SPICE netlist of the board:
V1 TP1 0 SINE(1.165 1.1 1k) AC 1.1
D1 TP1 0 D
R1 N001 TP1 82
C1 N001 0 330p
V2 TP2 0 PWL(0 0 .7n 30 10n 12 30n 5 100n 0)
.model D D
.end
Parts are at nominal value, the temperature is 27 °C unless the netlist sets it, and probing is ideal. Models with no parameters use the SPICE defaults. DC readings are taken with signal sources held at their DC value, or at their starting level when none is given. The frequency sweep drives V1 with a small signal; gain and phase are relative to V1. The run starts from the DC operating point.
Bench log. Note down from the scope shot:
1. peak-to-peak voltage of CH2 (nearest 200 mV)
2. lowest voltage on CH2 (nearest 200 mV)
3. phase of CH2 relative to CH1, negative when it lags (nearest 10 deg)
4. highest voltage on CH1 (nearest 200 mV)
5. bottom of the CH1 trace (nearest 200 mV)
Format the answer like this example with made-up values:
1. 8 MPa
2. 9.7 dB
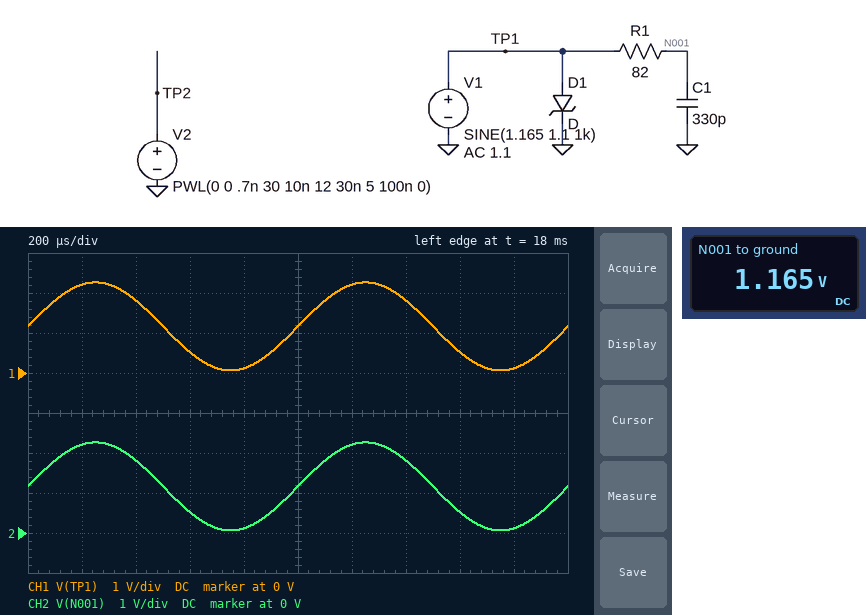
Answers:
1. 2.2 V
2. 0 V
3. 0 deg
4. 2.2 V
5. 0 V
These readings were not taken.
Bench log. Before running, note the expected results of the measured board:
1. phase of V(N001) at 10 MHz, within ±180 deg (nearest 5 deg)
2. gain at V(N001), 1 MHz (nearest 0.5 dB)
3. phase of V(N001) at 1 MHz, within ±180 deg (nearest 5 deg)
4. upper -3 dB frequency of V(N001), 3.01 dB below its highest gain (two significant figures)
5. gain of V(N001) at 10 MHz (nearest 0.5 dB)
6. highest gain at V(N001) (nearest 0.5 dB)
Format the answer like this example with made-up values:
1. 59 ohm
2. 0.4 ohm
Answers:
1. -60 deg
2. 0 dB
3. -10 deg
4. 5.9 MHz
5. -6.0 dB
6. 0 dB
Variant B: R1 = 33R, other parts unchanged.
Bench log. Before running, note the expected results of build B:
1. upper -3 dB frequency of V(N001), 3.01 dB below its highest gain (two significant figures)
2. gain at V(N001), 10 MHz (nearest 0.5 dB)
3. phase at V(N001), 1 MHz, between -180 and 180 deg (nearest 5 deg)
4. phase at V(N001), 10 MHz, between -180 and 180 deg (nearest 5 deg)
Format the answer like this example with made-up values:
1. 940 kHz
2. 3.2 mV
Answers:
1. 15 MHz
2. -1.5 dB
3. -5 deg
4. -35 deg
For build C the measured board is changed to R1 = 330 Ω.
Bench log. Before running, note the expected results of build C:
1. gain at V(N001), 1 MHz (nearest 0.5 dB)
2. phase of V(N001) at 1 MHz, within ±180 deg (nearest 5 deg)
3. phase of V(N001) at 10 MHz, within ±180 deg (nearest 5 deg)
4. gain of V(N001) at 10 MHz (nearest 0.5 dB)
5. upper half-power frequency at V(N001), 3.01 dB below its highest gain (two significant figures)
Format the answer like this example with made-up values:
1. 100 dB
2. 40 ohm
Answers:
1. -1.5 dB
2. -35 deg
3. -80 deg
4. -17.0 dB
5. 1.5 MHz
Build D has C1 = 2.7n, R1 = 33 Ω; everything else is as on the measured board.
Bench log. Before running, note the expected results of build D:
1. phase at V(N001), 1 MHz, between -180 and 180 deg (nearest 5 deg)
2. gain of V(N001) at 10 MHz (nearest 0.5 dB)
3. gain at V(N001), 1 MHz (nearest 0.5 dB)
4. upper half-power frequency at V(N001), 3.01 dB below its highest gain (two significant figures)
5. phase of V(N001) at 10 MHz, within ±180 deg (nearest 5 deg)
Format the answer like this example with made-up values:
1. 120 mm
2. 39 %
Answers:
1. -30 deg
2. -15.0 dB
3. -1.0 dB
4. 1.8 MHz
5. -80 deg
